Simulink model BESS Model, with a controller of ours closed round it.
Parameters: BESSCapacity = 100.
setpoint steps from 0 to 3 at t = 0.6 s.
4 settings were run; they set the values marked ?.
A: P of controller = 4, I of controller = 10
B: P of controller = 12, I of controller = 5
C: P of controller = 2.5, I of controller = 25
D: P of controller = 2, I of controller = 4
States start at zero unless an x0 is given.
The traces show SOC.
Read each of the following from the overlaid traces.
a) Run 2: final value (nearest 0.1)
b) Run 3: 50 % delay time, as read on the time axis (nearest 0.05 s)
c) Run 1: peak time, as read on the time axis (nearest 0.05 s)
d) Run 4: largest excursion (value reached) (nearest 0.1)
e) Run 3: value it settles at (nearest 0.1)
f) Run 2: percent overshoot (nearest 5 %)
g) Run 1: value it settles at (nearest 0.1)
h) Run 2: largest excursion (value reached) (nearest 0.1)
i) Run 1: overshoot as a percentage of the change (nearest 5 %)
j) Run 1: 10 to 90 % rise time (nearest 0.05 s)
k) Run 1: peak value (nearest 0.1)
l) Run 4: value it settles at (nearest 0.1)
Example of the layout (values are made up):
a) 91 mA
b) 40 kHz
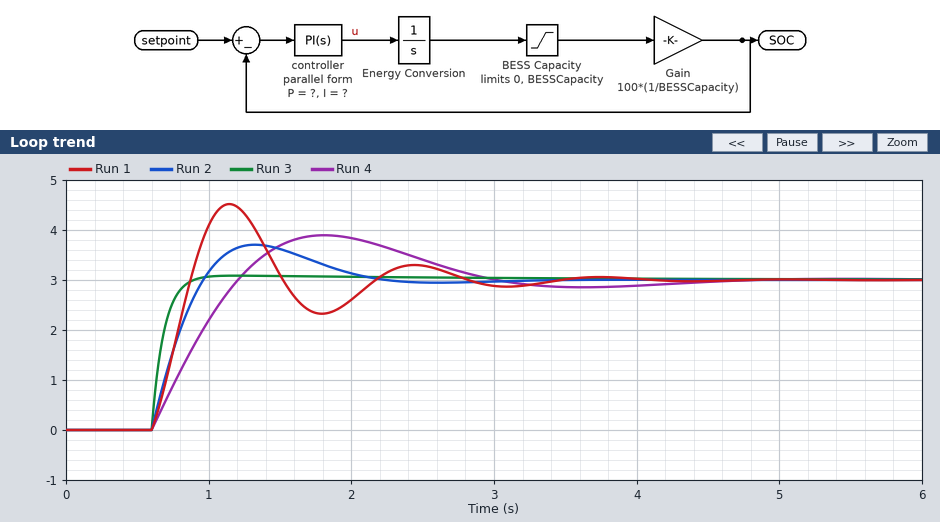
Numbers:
a) 3.0
b) 0.65 s
c) 1.15 s
d) 3.9
e) 3.0
f) 25 %
g) 3.0
h) 3.7
i) 50 %
j) 0.20 s
k) 4.5
l) 3.0
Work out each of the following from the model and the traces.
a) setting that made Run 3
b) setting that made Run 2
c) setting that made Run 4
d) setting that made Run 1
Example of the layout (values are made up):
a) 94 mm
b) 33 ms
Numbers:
a) B
b) A
c) D
d) C
